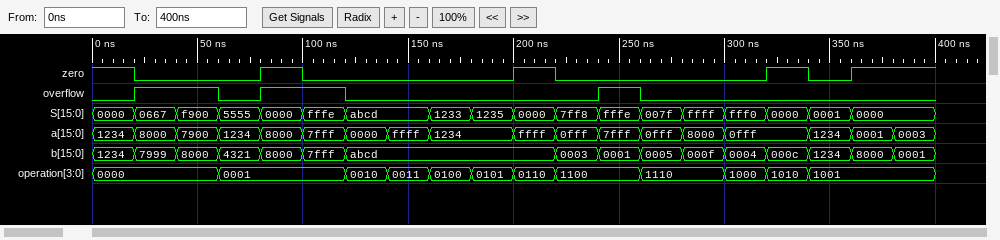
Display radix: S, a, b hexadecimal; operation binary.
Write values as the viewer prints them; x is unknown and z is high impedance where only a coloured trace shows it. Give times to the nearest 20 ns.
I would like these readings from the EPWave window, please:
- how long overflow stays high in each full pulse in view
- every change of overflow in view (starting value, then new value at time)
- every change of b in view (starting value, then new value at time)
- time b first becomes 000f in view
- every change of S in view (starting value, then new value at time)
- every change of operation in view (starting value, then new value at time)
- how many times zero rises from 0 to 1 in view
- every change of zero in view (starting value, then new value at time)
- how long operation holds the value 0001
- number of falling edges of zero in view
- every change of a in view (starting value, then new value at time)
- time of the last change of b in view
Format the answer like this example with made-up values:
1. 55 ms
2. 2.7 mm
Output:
1. 40 ns, 40 ns, 20 ns
2. 0, 1 at 20 ns, 0 at 60 ns, 1 at 80 ns, 0 at 120 ns, 1 at 240 ns, 0 at 260 ns
3. 1234, 7999 at 20 ns, 8000 at 40 ns, 4321 at 60 ns, 8000 at 80 ns, 7fff at 100 ns, abcd at 120 ns, 0003 at 220 ns, 0001 at 240 ns, 0005 at 260 ns, 000f at 280 ns, 0004 at 300 ns, 000c at 320 ns, 1234 at 340 ns, 8000 at 360 ns, 0001 at 380 ns
4. 280 ns
5. 0000, 0667 at 20 ns, f900 at 40 ns, 5555 at 60 ns, 0000 at 80 ns, fffe at 100 ns, abcd at 120 ns, 1233 at 160 ns, 1235 at 180 ns, 0000 at 200 ns, 7ff8 at 220 ns, fffe at 240 ns, 007f at 260 ns, ffff at 280 ns, fff0 at 300 ns, 0000 at 320 ns, 0001 at 340 ns, 0000 at 360 ns
6. 0000, 0001 at 60 ns, 0010 at 120 ns, 0011 at 140 ns, 0100 at 160 ns, 0101 at 180 ns, 0110 at 200 ns, 1100 at 220 ns, 1110 at 260 ns, 1000 at 300 ns, 1010 at 320 ns, 1001 at 340 ns
7. 4
8. 1, 0 at 20 ns, 1 at 80 ns, 0 at 100 ns, 1 at 200 ns, 0 at 220 ns, 1 at 320 ns, 0 at 340 ns, 1 at 360 ns
9. 60 ns
10. 4
11. 1234, 8000 at 20 ns, 7900 at 40 ns, 1234 at 60 ns, 8000 at 80 ns, 7fff at 100 ns, 0000 at 120 ns, ffff at 140 ns, 1234 at 160 ns, ffff at 200 ns, 0fff at 220 ns, 7fff at 240 ns, 0fff at 260 ns, 8000 at 280 ns, 0fff at 300 ns, 1234 at 340 ns, 0001 at 360 ns, 0003 at 380 ns
12. 380 ns
